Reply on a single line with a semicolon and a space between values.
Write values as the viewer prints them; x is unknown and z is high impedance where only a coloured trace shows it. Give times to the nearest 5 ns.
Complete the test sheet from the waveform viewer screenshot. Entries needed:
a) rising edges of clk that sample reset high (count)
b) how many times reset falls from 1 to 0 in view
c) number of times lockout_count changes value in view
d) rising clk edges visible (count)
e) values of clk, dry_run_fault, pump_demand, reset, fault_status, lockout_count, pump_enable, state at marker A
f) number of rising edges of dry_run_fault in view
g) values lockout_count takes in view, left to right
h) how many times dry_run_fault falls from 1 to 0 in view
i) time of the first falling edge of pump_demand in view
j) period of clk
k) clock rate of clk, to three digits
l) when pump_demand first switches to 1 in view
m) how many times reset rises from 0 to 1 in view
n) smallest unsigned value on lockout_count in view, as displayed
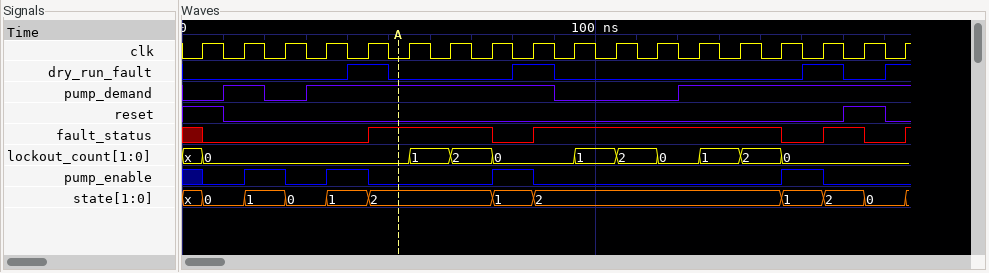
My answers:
2; 2; 10; 18; clk=0, dry_run_fault=0, pump_demand=1, reset=0, fault_status=1, lockout_count=0, pump_enable=0, state=2; 4; x, 0, 1, 2, 0, 1, 2, 0, 1, 2, 0; 3; 20 ns; 10 ns; 100 MHz; 10 ns; 1; 0
